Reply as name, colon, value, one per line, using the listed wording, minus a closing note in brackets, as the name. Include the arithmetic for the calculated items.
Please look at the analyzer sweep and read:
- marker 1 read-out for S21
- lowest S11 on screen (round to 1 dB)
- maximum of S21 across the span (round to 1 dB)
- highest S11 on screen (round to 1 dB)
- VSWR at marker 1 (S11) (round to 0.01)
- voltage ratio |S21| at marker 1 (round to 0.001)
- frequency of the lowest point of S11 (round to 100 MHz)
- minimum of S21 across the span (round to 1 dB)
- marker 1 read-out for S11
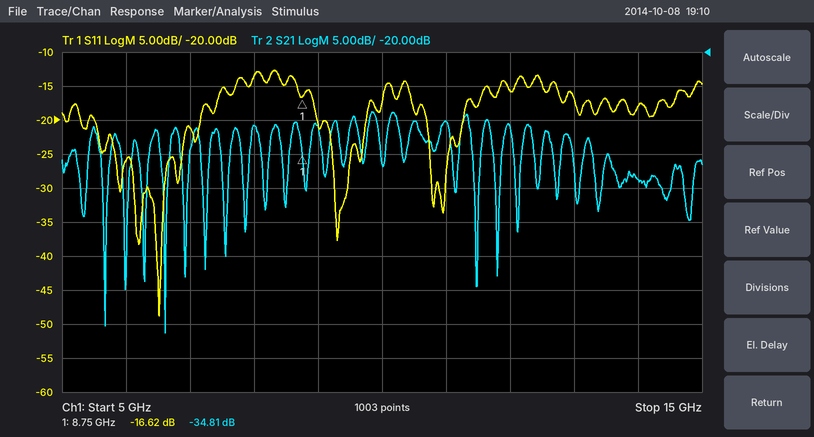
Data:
marker 1 read-out for S21: -34.81 dB
lowest S11 on screen: -49 dB
maximum of S21 across the span: -29 dB
highest S11 on screen: -13 dB
VSWR at marker 1 (S11): (1 + 0.1476)/(1 − 0.1476) ≈ 1.35
voltage ratio |S21| at marker 1: 10^(-34.81/20) ≈ 0.018
frequency of the lowest point of S11: 6.5 GHz
minimum of S21 across the span: -61 dB
marker 1 read-out for S11: -16.62 dB
